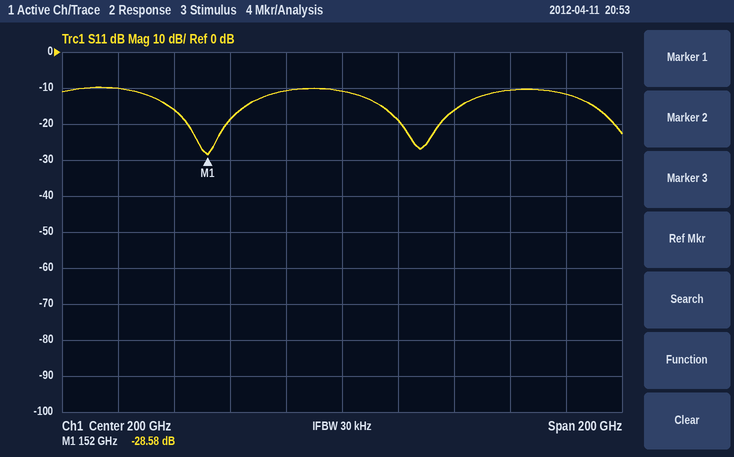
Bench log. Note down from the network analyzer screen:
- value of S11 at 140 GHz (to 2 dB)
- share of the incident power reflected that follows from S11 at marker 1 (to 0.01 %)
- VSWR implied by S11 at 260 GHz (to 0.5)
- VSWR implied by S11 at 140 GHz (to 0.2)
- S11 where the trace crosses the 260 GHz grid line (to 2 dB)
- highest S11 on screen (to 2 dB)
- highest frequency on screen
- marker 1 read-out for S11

-16 dB
0.14 %
2.0
1.4
-10 dB
-10 dB
300 GHz
-28.58 dB
